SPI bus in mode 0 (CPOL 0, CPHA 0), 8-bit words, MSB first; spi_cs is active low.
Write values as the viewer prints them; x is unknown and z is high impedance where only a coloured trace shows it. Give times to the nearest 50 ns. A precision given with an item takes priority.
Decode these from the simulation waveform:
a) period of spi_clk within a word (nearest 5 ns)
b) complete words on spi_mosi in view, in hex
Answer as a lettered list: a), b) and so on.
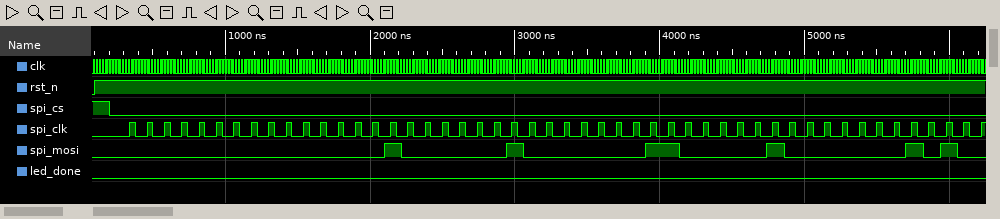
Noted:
a) 120 ns
b) 00, 01, 02, 03, 04, 05
